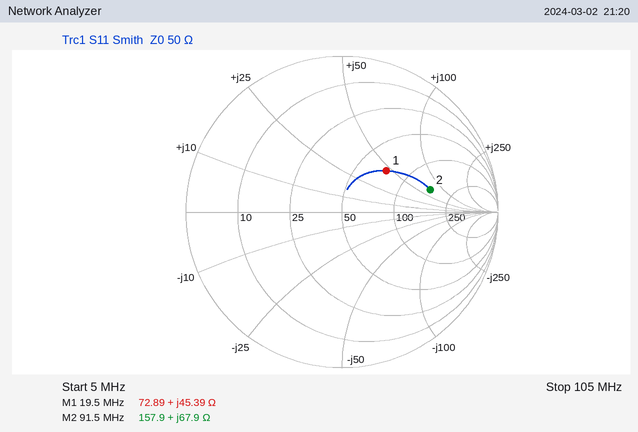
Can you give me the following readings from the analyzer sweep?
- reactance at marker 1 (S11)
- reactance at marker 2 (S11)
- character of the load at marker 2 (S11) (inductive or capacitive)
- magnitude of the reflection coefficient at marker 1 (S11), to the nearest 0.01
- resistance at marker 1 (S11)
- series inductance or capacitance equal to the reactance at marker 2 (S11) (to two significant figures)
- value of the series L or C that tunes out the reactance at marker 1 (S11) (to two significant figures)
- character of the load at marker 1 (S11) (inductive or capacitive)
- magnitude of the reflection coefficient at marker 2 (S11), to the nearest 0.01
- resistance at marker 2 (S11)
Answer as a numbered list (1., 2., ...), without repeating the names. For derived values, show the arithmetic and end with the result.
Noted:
1. +45.39 Ω
2. +67.9 Ω
3. inductive
4. 0.39
5. 72.89 Ω
6. L = 67.9 Ω/(2π × 91.5 MHz) ≈ 118 nH, so 120 nH to two significant figures
7. C = 1/(2π × 19.5 MHz × 45.39 Ω) ≈ 180 pF
8. inductive
9. 0.58
10. 157.9 Ω
